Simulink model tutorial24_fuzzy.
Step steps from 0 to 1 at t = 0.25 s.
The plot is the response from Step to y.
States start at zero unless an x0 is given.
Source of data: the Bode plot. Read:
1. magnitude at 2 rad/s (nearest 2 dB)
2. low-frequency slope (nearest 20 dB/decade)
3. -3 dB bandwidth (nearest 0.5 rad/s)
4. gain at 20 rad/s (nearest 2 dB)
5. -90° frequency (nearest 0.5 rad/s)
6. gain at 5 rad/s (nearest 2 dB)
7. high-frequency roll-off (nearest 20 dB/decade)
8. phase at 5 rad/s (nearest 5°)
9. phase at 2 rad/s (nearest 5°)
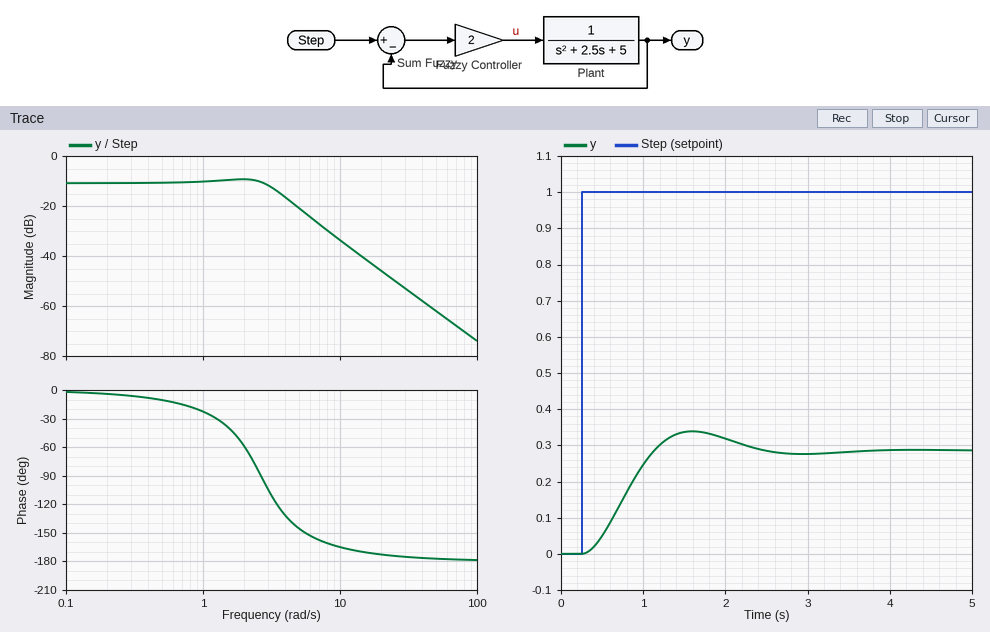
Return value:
-10 dB
0 dB/decade
3.5 rad/s
-46 dB
2.5 rad/s
-20 dB
-40 dB/decade
-145°
-60°
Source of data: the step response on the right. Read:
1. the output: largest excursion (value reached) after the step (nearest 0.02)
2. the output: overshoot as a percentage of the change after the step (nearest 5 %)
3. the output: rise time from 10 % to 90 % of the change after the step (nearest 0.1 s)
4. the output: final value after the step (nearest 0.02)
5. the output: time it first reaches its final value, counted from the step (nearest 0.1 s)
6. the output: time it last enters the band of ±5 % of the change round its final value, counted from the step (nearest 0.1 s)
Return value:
0.34
20 %
0.6 s
0.28
0.9 s
2.0 s
